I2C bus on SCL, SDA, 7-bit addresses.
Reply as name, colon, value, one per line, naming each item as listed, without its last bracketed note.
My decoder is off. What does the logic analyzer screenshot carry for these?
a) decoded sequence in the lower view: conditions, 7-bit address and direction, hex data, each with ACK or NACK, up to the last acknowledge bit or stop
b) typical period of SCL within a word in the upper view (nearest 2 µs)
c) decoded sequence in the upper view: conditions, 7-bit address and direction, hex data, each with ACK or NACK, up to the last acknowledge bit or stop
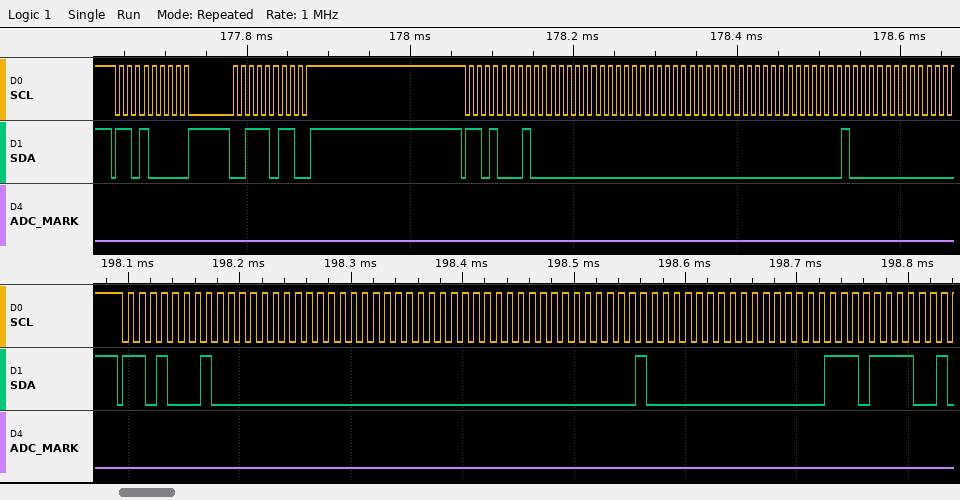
decoded sequence in the lower view: conditions, 7-bit address and direction, hex data, each with ACK or NACK, up to the last acknowledge bit or stop: start, address 68 read ACK, 00 ACK, 00 ACK, 00 ACK, 00 ACK, 40 ACK, 00 ACK, EF ACK
typical period of SCL within a word in the upper view: 10 µs
decoded sequence in the upper view: conditions, 7-bit address and direction, hex data, each with ACK or NACK, up to the last acknowledge bit or stop: start, address 68 write ACK, 3B ACK, stop, start, address 68 read ACK, 00 ACK, 00 ACK, 00 ACK, 00 ACK, 40 ACK
